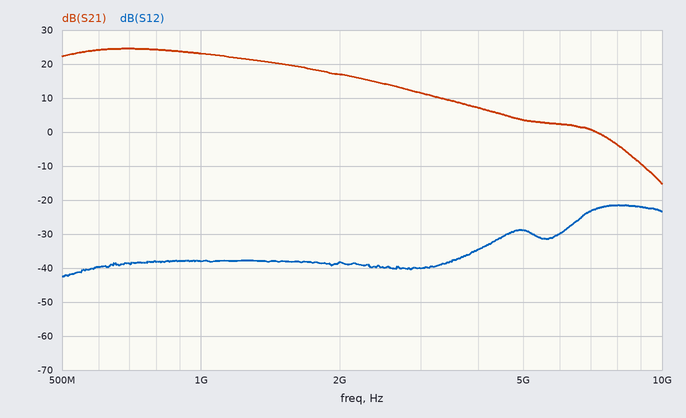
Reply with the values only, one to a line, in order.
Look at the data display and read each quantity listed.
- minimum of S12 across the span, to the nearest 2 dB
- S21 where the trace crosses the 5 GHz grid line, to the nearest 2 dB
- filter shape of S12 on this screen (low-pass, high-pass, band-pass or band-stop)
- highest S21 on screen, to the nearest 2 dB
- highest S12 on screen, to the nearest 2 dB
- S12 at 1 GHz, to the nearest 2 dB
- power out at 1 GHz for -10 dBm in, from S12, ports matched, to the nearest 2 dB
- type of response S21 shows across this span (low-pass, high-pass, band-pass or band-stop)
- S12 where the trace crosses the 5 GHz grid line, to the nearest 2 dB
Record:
-42 dB
4 dB
high-pass
24 dB
-22 dB
-38 dB
-48 dBm
low-pass
-28 dB
